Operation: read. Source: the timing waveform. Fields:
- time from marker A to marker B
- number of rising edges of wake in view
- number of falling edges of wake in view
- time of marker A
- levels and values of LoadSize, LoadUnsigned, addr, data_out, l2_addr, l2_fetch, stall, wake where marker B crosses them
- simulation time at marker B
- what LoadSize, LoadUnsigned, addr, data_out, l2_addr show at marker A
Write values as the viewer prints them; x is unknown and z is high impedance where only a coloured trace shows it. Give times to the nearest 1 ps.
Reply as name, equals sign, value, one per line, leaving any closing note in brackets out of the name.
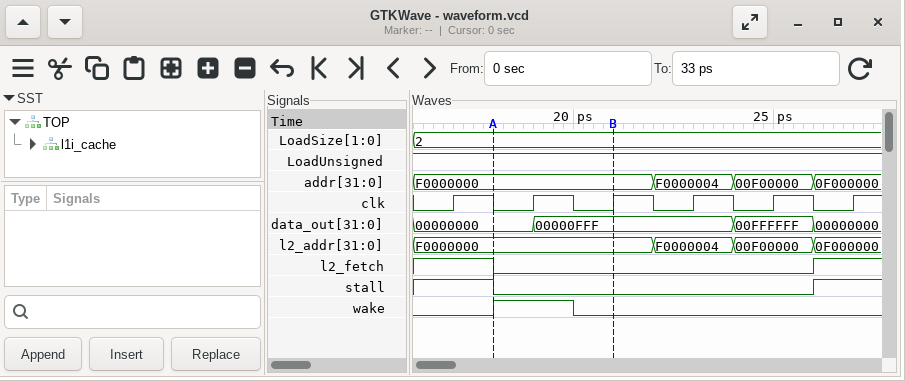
time from marker A to marker B = 3 ps
number of rising edges of wake in view = 1
number of falling edges of wake in view = 1
time of marker A = 18 ps
levels and values of LoadSize, LoadUnsigned, addr, data_out, l2_addr, l2_fetch, stall, wake where marker B crosses them = LoadSize=2, LoadUnsigned=1, addr=F0000000, data_out=00000FFF, l2_addr=F0000000, l2_fetch=0, stall=0, wake=0
simulation time at marker B = 21 ps
what LoadSize, LoadUnsigned, addr, data_out, l2_addr show at marker A = LoadSize=2, LoadUnsigned=1, addr=F0000000, data_out=00000000, l2_addr=F0000000
